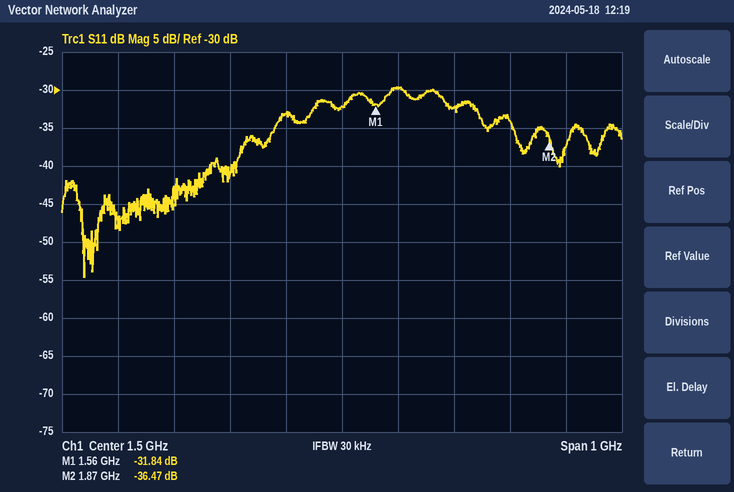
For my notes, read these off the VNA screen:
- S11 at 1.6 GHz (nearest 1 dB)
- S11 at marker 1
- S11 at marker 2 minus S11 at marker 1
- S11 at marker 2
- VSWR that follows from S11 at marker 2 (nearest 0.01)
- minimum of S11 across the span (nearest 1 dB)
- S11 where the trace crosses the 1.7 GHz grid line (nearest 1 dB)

-30 dB
-31.84 dB
-4.63 dB
-36.47 dB
1.03
-55 dB
-32 dB
